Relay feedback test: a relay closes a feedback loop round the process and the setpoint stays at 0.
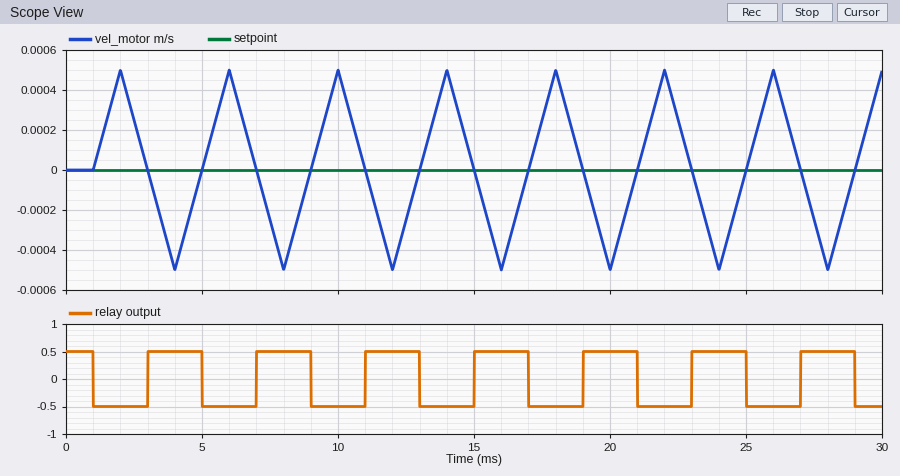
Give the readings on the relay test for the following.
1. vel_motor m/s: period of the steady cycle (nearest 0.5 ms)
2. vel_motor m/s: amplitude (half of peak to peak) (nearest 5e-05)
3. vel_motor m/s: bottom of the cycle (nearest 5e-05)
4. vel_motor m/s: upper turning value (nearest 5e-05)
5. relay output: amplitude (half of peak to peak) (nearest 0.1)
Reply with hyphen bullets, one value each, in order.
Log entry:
- 4.0 ms
- 0.00050
- -0.00050
- 0.00050
- 0.5
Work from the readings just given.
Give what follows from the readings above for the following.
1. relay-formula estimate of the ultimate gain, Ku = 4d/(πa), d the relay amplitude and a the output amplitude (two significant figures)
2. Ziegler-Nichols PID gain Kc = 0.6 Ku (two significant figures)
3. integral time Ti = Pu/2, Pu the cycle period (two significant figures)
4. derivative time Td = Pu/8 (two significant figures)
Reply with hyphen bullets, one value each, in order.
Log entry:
- 1300
- 780
- 2.0 ms
- 0.50 ms
